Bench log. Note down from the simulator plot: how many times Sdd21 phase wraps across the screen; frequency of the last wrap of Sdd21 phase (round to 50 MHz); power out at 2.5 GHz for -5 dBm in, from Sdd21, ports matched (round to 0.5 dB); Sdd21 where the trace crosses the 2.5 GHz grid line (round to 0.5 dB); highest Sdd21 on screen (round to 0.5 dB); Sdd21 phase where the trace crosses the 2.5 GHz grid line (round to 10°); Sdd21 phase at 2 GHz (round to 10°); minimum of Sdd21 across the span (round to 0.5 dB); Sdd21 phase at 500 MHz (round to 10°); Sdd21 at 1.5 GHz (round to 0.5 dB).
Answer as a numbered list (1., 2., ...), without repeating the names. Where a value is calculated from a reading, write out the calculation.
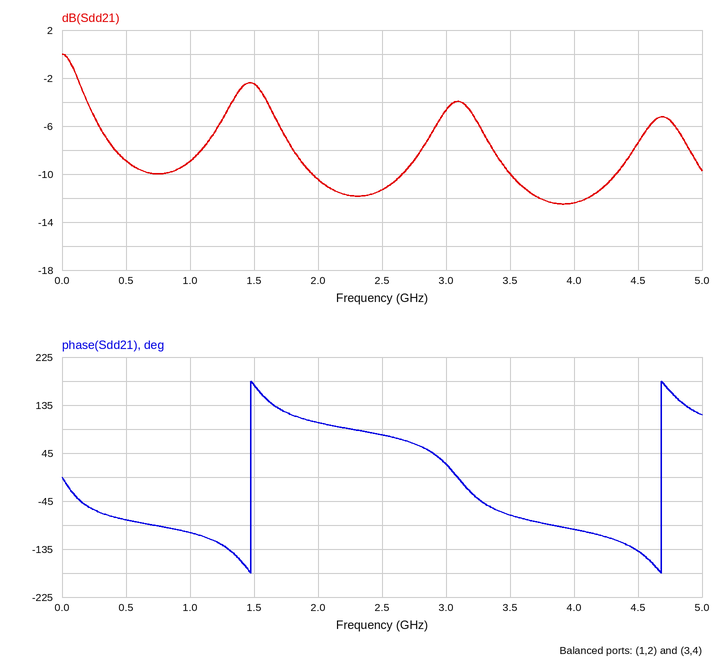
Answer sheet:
1. 2
2. 4.70 GHz
3. -5 dBm + (-11.5 dB) = -16.5 dBm
4. -11.5 dB
5. 0.0 dB
6. 80°
7. 100°
8. -12.5 dB
9. -80°
10. -2.5 dB
